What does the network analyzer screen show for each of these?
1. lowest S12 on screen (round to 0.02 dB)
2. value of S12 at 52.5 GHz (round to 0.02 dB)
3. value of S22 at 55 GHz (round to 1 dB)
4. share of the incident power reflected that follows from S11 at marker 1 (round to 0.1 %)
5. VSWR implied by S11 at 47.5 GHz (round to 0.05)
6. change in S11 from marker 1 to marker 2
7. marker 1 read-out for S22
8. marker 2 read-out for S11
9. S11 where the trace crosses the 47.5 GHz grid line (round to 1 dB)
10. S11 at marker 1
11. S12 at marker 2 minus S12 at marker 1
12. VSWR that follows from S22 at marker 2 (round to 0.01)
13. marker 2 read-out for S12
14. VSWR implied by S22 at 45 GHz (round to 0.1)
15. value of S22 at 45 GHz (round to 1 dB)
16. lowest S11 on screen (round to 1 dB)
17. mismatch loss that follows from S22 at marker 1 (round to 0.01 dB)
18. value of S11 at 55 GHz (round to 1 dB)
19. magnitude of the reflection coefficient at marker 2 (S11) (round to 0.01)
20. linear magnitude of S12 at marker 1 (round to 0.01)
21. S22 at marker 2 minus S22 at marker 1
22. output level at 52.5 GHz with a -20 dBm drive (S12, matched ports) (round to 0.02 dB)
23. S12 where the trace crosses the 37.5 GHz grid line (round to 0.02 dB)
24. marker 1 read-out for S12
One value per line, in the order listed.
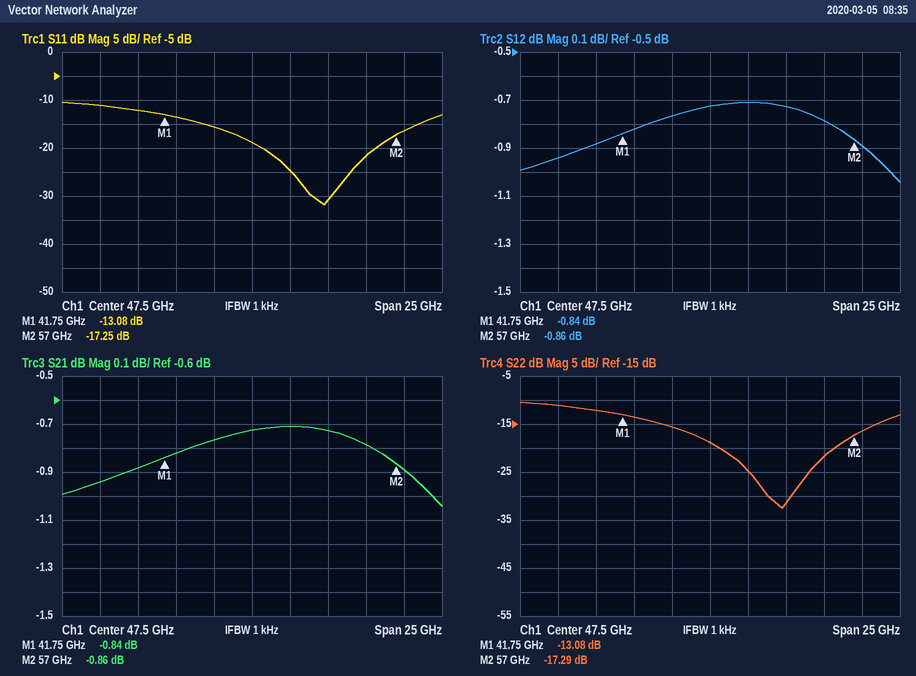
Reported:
-1.04 dB
-0.72 dB
-22 dB
4.9 %
1.25
-4.17 dB
-13.08 dB
-17.25 dB
-19 dB
-13.08 dB
-0.02 dB
1.32
-0.86 dB
1.4
-16 dB
-32 dB
0.22 dB
-22 dB
0.14
0.91
-4.21 dB
-20.72 dBm
-0.94 dB
-0.84 dB
